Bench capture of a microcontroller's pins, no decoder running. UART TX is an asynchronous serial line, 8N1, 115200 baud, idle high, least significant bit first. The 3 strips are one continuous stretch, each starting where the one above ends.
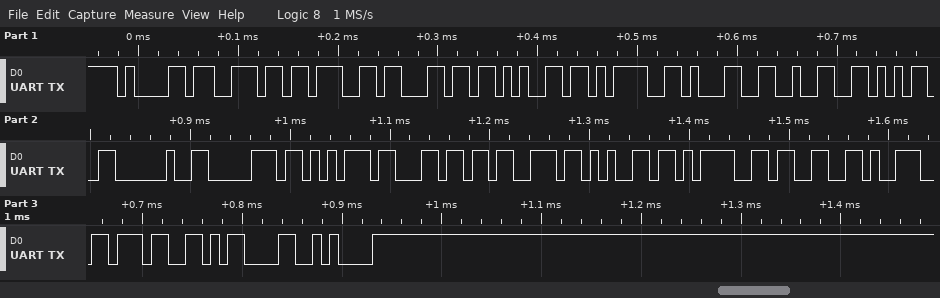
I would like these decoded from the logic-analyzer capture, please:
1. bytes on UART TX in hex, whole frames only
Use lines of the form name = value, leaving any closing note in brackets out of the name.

bytes on UART TX in hex, whole frames only = 61 6E 67 6C 65 3D 31 32 35 20 70 75 6C 73 65 3D 33 39 37 0D 0A
